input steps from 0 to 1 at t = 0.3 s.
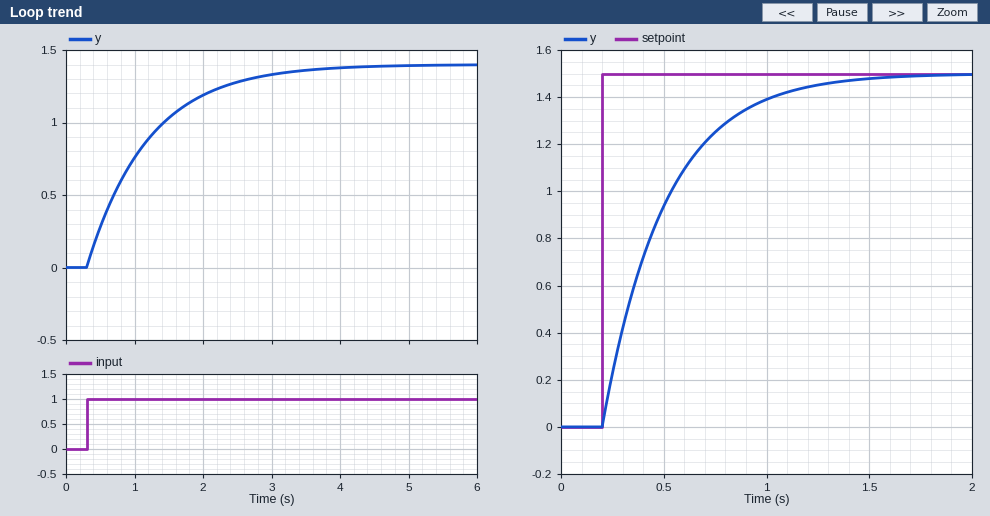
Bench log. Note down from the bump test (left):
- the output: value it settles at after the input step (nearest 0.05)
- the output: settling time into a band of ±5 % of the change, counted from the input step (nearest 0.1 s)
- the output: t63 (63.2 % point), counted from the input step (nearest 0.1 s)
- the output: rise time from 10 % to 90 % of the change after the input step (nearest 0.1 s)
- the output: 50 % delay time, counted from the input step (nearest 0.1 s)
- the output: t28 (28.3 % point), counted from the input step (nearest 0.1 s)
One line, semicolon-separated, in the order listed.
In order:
1.40; 2.7 s; 0.9 s; 2.0 s; 0.6 s; 0.3 s
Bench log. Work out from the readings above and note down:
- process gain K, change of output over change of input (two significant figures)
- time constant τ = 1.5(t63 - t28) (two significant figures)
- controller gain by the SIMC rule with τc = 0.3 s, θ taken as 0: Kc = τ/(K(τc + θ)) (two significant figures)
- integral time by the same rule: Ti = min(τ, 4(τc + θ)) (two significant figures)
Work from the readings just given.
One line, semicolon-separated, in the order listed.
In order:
1.4; 0.90 s; 2.1; 0.90 s
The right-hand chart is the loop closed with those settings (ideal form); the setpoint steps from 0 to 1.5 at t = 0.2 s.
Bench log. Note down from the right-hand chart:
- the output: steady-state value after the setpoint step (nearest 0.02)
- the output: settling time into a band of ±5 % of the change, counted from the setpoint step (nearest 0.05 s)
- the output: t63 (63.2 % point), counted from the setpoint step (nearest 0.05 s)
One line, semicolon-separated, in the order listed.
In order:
1.50; 0.90 s; 0.30 s
